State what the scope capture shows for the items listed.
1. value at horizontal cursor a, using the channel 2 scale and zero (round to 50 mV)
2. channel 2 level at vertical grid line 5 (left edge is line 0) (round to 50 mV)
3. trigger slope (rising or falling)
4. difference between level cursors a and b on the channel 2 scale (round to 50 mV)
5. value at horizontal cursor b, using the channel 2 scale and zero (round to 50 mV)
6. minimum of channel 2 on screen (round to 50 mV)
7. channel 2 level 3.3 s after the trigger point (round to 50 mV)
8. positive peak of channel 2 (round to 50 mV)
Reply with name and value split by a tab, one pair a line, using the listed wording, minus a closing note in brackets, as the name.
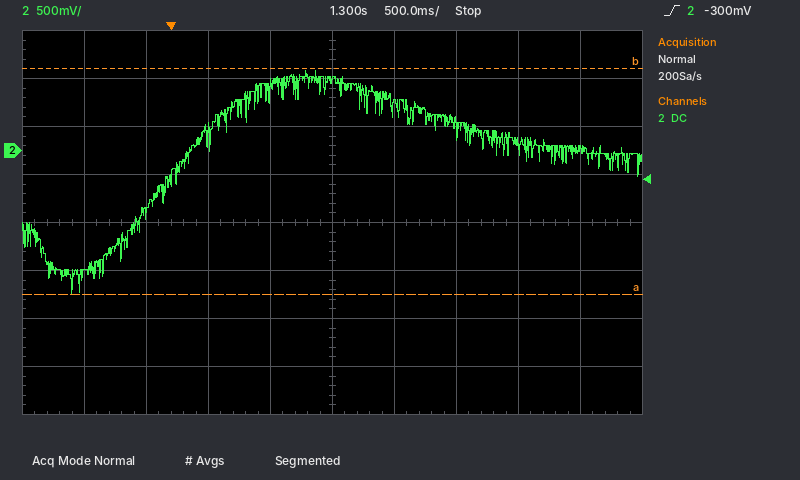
value at horizontal cursor a, using the channel 2 scale and zero	-1.50 V
channel 2 level at vertical grid line 5 (left edge is line 0)	750 mV
trigger slope	rising
difference between level cursors a and b on the channel 2 scale	2.35 V
value at horizontal cursor b, using the channel 2 scale and zero	850 mV
minimum of channel 2 on screen	-1.50 V
channel 2 level 3.3 s after the trigger point	0 mV
positive peak of channel 2	850 mV
